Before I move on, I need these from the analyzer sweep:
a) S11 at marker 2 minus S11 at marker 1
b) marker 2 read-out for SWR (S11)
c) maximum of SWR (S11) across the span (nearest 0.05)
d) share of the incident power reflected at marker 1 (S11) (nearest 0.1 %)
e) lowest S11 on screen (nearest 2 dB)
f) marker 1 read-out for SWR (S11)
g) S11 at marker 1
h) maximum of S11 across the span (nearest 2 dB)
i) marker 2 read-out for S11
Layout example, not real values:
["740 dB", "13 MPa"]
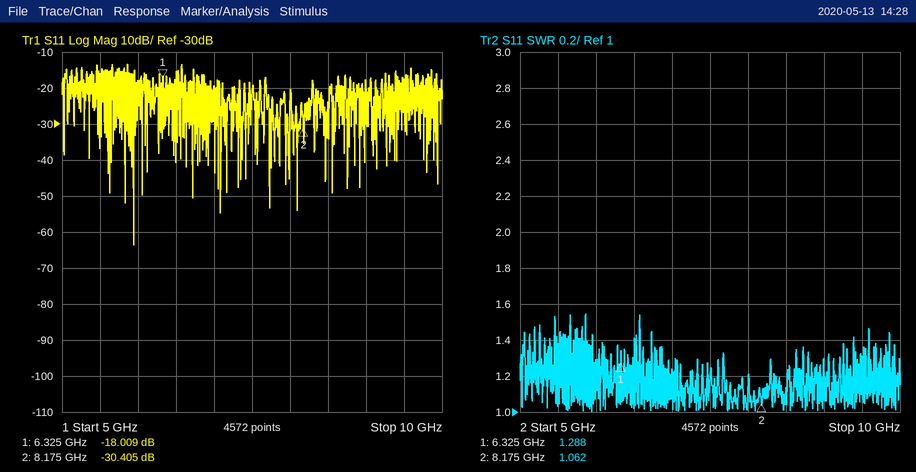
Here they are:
["-12.396 dB", "1.062", "1.55", "1.6 %", "-64 dB", "1.288", "-18.009 dB", "-14 dB", "-30.405 dB"]
